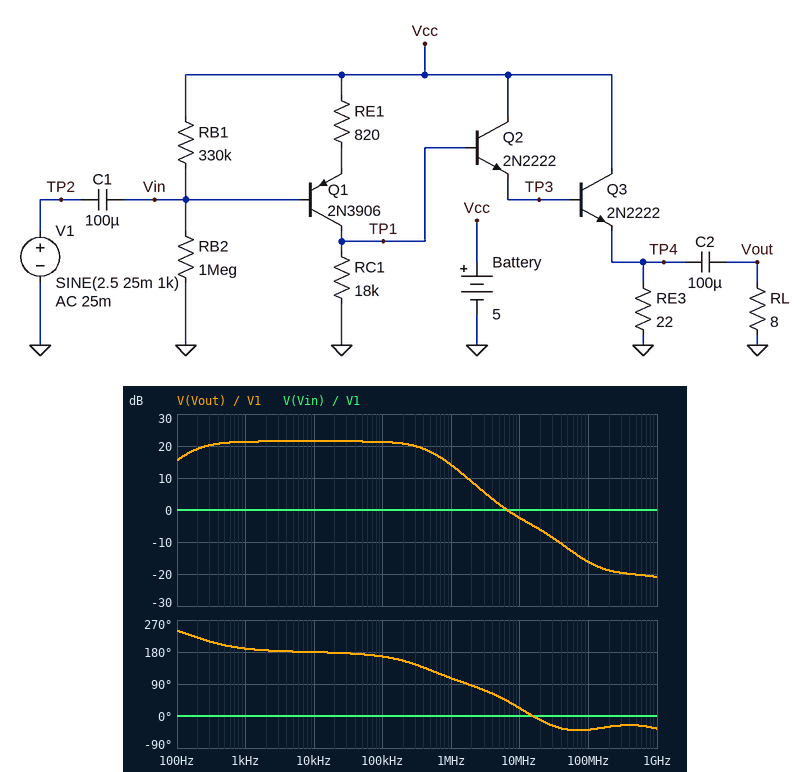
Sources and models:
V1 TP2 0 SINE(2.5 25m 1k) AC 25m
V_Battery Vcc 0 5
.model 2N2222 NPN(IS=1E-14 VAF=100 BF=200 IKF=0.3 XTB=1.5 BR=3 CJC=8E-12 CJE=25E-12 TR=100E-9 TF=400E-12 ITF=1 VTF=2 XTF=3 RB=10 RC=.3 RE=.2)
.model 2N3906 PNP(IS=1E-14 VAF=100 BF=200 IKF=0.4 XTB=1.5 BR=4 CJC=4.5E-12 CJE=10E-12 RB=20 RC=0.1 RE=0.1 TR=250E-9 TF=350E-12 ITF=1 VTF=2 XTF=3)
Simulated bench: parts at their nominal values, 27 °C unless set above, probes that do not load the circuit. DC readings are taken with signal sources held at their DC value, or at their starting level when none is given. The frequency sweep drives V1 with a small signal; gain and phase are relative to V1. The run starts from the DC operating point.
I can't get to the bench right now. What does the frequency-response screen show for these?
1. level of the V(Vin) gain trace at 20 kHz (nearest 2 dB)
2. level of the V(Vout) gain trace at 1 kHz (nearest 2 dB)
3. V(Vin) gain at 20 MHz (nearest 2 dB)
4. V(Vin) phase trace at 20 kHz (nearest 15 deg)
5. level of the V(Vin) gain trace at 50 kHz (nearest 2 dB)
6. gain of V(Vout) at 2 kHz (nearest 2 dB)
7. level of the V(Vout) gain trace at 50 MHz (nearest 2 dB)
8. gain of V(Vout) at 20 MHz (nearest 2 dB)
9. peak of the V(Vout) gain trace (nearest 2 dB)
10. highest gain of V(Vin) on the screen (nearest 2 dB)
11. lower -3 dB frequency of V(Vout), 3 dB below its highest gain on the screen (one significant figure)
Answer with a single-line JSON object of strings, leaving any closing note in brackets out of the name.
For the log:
{"level of the V(Vin) gain trace at 20 kHz": "0 dB", "level of the V(Vout) gain trace at 1 kHz": "22 dB", "V(Vin) gain at 20 MHz": "0 dB", "V(Vin) phase trace at 20 kHz": "0 deg", "level of the V(Vin) gain trace at 50 kHz": "0 dB", "gain of V(Vout) at 2 kHz": "22 dB", "level of the V(Vout) gain trace at 50 MHz": "-12 dB", "gain of V(Vout) at 20 MHz": "-6 dB", "peak of the V(Vout) gain trace": "22 dB", "highest gain of V(Vin) on the screen": "0 dB", "lower -3 dB frequency of V(Vout), 3 dB below its highest gain on the screen": "200 Hz"}
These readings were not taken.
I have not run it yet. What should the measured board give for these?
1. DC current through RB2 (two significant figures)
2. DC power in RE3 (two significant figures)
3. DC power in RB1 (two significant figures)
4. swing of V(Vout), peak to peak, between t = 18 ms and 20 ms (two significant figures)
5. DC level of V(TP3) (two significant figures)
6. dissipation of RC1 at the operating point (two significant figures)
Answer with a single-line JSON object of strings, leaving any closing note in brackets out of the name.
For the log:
{"DC current through RB2": "4.2 µA", "DC power in RE3": "450 mW", "DC power in RB1": "2.1 µW", "swing of V(Vout), peak to peak, between t = 18 ms and 20 ms": "470 mV", "DC level of V(TP3)": "4.0 V", "dissipation of RC1 at the operating point": "1.2 mW"}
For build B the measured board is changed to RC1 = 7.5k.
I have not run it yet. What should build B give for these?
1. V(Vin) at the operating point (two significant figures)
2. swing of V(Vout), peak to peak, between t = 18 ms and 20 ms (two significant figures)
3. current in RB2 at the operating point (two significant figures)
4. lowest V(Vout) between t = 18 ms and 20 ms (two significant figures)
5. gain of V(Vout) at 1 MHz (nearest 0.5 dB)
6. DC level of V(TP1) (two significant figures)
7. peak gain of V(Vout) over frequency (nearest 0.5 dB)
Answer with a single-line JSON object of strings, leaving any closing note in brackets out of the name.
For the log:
{"V(Vin) at the operating point": "4.1 V", "swing of V(Vout), peak to peak, between t = 18 ms and 20 ms": "300 mV", "current in RB2 at the operating point": "4.1 µA", "lowest V(Vout) between t = 18 ms and 20 ms": "-140 mV", "gain of V(Vout) at 1 MHz": "15.0 dB", "DC level of V(TP1)": "2.3 V", "peak gain of V(Vout) over frequency": "16.0 dB"}
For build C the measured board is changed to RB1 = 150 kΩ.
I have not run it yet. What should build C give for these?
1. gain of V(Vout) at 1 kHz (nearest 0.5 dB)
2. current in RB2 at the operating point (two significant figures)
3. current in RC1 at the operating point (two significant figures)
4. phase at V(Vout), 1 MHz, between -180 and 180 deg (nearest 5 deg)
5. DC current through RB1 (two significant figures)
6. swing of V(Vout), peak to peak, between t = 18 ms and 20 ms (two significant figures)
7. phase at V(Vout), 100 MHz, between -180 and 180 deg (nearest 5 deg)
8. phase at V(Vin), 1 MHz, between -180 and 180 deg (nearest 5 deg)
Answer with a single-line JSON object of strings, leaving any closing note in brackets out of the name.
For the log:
{"gain of V(Vout) at 1 kHz": "-37.5 dB", "current in RB2 at the operating point": "4.4 µA", "current in RC1 at the operating point": "51 µA", "phase at V(Vout), 1 MHz, between -180 and 180 deg": "140 deg", "DC current through RB1": "4.1 µA", "swing of V(Vout), peak to peak, between t = 18 ms and 20 ms": "25 mV", "phase at V(Vout), 100 MHz, between -180 and 180 deg": "85 deg", "phase at V(Vin), 1 MHz, between -180 and 180 deg": "0 deg"}
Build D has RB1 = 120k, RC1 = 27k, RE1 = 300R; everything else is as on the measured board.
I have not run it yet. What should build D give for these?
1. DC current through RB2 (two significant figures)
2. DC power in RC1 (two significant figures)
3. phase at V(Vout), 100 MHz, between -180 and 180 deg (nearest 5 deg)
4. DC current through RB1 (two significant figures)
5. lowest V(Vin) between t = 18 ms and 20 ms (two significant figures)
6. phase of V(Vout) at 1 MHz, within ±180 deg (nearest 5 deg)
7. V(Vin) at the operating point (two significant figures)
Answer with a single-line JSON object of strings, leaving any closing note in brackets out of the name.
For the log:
{"DC current through RB2": "4.5 µA", "DC power in RC1": "1.7 µW", "phase at V(Vout), 100 MHz, between -180 and 180 deg": "85 deg", "DC current through RB1": "4.4 µA", "lowest V(Vin) between t = 18 ms and 20 ms": "4.4 V", "phase of V(Vout) at 1 MHz, within ±180 deg": "-170 deg", "V(Vin) at the operating point": "4.5 V"}
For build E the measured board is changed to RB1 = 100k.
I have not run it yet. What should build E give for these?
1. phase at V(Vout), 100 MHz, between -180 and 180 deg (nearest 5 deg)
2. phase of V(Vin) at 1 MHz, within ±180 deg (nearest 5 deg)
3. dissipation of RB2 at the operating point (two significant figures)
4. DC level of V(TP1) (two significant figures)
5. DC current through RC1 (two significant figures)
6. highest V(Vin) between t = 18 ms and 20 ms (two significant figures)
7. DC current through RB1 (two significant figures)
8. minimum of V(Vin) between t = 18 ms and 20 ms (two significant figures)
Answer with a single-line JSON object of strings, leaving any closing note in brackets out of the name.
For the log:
{"phase at V(Vout), 100 MHz, between -180 and 180 deg": "85 deg", "phase of V(Vin) at 1 MHz, within ±180 deg": "0 deg", "dissipation of RB2 at the operating point": "21 µW", "DC level of V(TP1)": "7.9 mV", "DC current through RC1": "440 nA", "highest V(Vin) between t = 18 ms and 20 ms": "4.6 V", "DC current through RB1": "4.5 µA", "minimum of V(Vin) between t = 18 ms and 20 ms": "4.5 V"}
